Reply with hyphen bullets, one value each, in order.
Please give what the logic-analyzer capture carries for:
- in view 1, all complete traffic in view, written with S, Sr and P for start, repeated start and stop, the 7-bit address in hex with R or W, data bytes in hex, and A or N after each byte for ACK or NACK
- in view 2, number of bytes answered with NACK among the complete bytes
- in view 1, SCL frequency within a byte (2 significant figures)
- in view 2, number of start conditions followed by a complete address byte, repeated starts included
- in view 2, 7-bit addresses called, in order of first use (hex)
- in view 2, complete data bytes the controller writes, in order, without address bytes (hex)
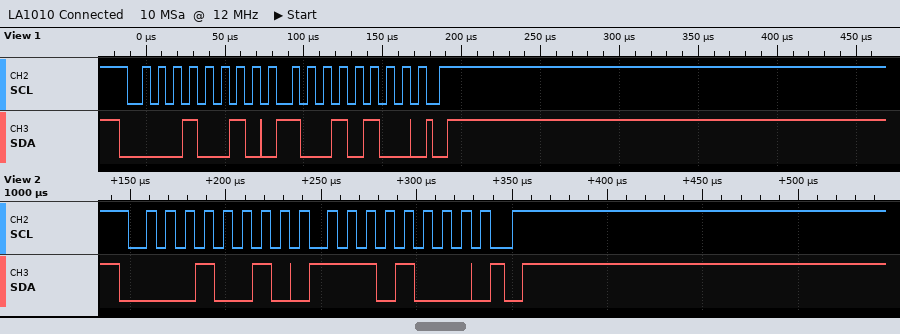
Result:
- S 09W A 94 A P
- 0
- 100 kHz
- 1
- 0x09
- E8
